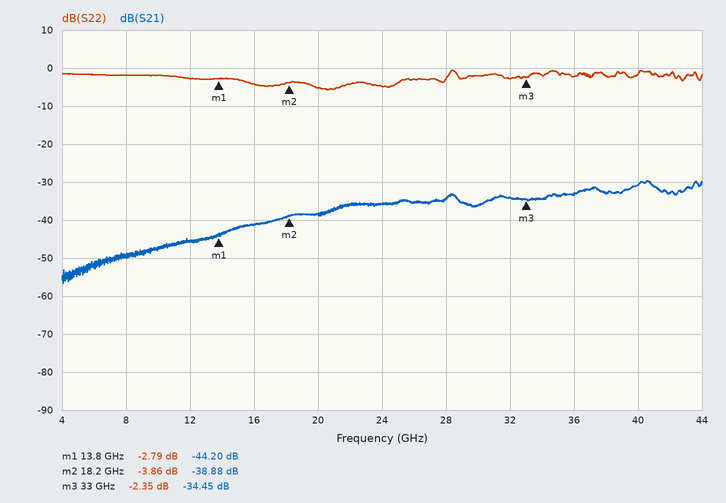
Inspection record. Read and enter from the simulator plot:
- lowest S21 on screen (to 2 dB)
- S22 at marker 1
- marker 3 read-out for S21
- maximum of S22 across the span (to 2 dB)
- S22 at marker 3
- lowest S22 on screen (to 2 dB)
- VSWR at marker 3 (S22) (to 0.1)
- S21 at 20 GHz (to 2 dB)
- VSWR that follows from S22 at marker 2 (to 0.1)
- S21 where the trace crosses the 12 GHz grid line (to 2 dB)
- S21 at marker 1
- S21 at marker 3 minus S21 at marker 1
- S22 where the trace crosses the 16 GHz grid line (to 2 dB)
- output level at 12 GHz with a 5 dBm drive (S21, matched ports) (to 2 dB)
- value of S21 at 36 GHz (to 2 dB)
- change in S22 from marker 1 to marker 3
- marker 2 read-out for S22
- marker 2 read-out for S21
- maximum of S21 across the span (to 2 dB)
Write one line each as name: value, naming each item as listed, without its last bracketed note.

lowest S21 on screen: -56 dB
S22 at marker 1: -2.79 dB
marker 3 read-out for S21: -34.45 dB
maximum of S22 across the span: 0 dB
S22 at marker 3: -2.35 dB
lowest S22 on screen: -6 dB
VSWR at marker 3 (S22): 7.4
S21 at 20 GHz: -38 dB
VSWR that follows from S22 at marker 2: 4.6
S21 where the trace crosses the 12 GHz grid line: -46 dB
S21 at marker 1: -44.20 dB
S21 at marker 3 minus S21 at marker 1: 9.75 dB
S22 where the trace crosses the 16 GHz grid line: -4 dB
output level at 12 GHz with a 5 dBm drive (S21, matched ports): -40 dBm
value of S21 at 36 GHz: -34 dB
change in S22 from marker 1 to marker 3: 0.44 dB
marker 2 read-out for S22: -3.86 dB
marker 2 read-out for S21: -38.88 dB
maximum of S21 across the span: -30 dB
